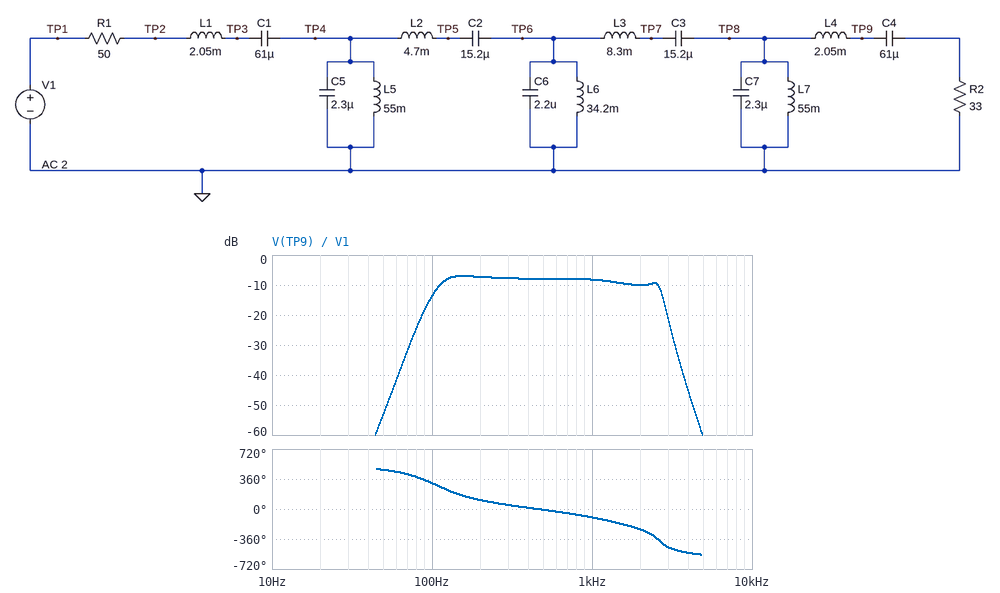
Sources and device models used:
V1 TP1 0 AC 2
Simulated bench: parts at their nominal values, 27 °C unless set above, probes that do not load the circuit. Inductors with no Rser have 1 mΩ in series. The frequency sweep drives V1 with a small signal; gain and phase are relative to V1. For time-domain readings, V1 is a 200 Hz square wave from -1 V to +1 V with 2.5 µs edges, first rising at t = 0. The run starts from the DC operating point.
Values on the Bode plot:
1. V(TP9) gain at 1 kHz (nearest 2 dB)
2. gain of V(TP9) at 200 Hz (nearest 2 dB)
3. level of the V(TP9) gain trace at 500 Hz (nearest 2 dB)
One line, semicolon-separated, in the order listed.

-8 dB; -8 dB; -8 dB
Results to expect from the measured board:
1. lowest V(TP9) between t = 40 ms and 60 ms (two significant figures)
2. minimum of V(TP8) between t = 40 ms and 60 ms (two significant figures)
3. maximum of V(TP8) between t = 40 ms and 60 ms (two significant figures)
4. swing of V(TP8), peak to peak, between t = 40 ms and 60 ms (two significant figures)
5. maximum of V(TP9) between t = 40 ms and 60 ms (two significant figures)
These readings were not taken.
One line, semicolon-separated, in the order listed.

-770 mV; -810 mV; 810 mV; 1.6 V; 770 mV
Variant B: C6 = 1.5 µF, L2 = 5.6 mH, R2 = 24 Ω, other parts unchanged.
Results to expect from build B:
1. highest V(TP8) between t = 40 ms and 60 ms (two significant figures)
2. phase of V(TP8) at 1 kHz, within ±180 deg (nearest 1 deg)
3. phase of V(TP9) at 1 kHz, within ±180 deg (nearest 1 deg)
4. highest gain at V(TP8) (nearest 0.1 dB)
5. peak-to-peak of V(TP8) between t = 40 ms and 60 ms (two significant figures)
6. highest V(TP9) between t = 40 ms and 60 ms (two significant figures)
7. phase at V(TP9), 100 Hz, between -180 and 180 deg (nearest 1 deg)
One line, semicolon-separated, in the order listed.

750 mV; -69 deg; -99 deg; -4.5 dB; 1.5 V; 690 mV; -65 deg
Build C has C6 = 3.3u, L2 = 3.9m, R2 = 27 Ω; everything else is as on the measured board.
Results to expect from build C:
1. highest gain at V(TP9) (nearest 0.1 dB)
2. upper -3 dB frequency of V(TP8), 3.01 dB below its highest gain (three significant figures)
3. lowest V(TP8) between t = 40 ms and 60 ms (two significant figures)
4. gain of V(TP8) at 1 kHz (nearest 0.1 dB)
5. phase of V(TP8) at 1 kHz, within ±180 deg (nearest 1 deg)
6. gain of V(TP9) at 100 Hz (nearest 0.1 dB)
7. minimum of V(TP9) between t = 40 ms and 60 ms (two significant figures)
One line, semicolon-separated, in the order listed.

-7.6 dB; 2.61 kHz; -740 mV; -8.6 dB; -85 deg; -14.1 dB; -700 mV
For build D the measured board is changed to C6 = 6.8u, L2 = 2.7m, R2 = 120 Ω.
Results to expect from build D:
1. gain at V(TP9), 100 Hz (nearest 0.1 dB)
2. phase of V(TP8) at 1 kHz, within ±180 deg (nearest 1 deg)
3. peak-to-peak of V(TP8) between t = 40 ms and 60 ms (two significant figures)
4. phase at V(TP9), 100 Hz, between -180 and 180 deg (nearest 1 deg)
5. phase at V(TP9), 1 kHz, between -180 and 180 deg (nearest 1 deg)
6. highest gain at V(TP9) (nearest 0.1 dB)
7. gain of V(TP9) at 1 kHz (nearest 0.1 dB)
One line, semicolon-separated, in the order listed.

-9.8 dB; -103 deg; 1.9 V; 6 deg; -109 deg; -2.1 dB; -6.3 dB
